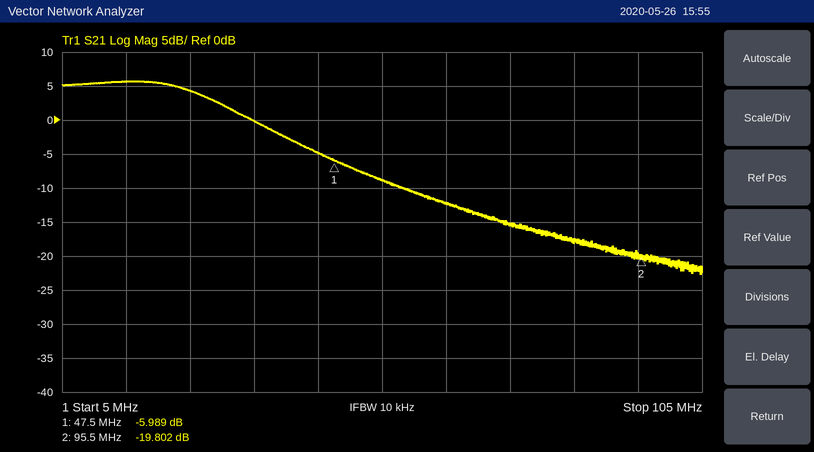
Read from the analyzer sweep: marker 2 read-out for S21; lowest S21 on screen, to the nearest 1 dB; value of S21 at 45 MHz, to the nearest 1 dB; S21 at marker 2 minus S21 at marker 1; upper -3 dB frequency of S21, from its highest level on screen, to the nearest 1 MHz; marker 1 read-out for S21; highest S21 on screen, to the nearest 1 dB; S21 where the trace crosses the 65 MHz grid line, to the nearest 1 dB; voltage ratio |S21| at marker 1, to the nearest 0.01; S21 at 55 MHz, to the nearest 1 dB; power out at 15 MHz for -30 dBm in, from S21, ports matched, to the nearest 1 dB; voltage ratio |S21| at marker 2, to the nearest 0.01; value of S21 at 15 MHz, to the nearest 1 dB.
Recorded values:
-19.802 dB
-23 dB
-5 dB
-13.813 dB
29 MHz
-5.989 dB
6 dB
-12 dB
0.50
-9 dB
-24 dBm
0.10
6 dB
